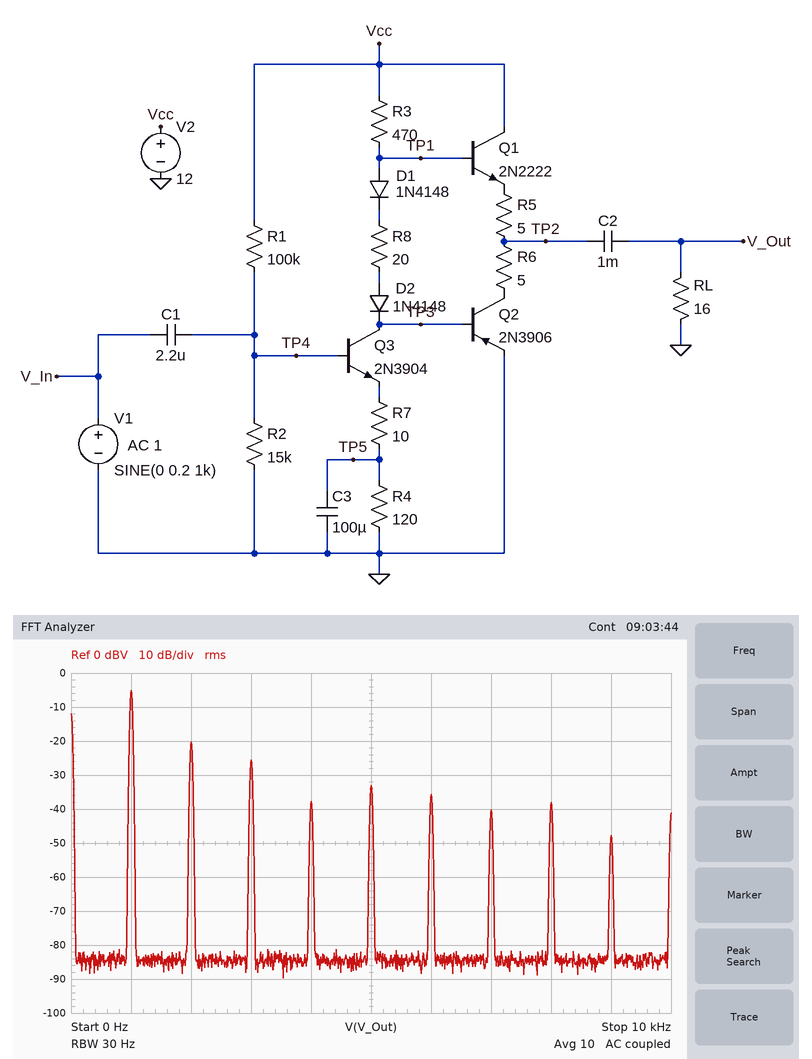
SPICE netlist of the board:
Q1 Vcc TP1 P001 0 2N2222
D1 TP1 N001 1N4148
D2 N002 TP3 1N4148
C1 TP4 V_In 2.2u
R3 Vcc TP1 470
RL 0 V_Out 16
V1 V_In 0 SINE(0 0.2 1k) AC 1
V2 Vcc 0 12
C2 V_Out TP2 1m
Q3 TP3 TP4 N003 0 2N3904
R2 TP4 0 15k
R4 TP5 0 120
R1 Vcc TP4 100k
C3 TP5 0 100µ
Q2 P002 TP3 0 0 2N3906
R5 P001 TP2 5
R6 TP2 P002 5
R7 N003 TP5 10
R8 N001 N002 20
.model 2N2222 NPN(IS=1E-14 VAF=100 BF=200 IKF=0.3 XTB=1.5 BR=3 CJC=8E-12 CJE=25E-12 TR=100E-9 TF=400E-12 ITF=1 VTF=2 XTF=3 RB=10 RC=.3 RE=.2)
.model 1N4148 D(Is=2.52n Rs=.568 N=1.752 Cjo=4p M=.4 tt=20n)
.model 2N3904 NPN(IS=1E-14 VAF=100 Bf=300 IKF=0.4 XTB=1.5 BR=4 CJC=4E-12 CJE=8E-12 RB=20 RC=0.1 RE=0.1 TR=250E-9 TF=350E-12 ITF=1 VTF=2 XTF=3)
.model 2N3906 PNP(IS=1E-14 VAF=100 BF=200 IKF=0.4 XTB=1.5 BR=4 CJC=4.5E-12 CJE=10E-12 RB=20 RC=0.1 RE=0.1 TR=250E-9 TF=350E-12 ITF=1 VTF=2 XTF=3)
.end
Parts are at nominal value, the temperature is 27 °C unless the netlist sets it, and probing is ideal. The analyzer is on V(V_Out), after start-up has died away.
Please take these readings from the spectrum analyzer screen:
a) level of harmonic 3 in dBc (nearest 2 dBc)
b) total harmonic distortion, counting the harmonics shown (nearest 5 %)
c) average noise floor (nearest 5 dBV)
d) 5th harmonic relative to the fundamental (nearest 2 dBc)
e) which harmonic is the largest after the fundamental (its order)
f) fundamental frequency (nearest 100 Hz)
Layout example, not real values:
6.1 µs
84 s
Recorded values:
-20 dBc
20 %
-85 dBV
-28 dBc
2
1.0 kHz
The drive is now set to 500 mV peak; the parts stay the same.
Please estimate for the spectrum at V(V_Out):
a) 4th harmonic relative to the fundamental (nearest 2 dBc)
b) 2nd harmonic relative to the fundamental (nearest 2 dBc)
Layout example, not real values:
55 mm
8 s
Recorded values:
-22 dBc
-6 dBc
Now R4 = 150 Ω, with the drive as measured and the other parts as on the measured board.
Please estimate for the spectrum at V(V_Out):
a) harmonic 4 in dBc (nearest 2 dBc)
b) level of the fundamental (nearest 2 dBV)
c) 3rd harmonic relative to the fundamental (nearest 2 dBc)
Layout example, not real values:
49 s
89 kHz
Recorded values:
-52 dBc
-6 dBV
-22 dBc
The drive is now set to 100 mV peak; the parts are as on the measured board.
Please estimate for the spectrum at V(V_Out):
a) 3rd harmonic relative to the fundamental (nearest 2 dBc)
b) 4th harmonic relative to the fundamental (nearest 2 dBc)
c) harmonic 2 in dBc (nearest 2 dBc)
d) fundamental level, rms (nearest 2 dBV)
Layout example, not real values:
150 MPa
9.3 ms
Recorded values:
-32 dBc
-26 dBc
-18 dBc
-8 dBV
